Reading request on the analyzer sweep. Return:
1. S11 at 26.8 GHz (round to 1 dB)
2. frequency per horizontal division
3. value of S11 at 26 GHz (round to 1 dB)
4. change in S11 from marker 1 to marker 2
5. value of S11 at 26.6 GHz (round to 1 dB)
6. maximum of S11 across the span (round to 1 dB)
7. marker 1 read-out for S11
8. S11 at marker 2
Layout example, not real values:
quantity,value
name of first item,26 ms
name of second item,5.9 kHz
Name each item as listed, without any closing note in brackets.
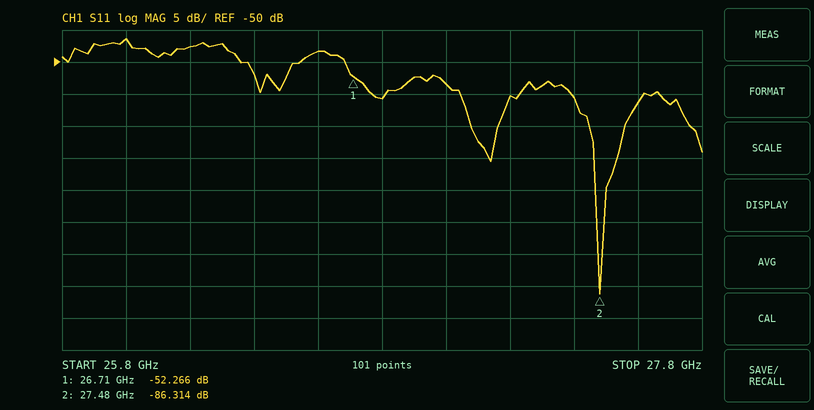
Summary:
quantity,value
S11 at 26.8 GHz,-56 dB
frequency per horizontal division,200 MHz
value of S11 at 26 GHz,-46 dB
change in S11 from marker 1 to marker 2,-34.048 dB
value of S11 at 26.6 GHz,-48 dB
maximum of S11 across the span,-46 dB
marker 1 read-out for S11,-52.266 dB
S11 at marker 2,-86.314 dB
